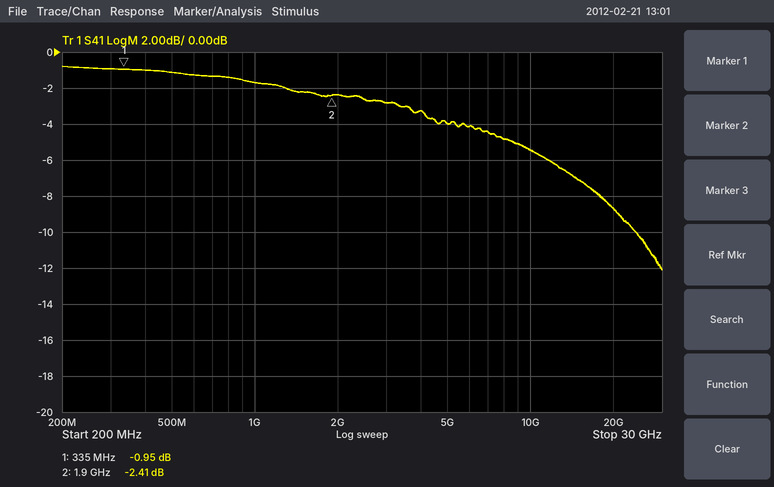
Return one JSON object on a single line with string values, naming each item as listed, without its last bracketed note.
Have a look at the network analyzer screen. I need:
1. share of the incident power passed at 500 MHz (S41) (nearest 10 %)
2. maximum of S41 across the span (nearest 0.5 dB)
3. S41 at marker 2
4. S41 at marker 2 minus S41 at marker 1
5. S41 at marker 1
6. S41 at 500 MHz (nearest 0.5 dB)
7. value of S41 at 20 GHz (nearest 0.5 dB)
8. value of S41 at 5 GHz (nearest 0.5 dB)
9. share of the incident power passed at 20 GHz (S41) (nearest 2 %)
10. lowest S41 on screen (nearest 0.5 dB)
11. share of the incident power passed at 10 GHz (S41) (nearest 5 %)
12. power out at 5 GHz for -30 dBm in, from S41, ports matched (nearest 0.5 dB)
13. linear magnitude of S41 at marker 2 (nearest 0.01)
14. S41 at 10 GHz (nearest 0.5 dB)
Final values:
{"share of the incident power passed at 500 MHz (S41)": "80 %", "maximum of S41 across the span": "-1.0 dB", "S41 at marker 2": "-2.41 dB", "S41 at marker 2 minus S41 at marker 1": "-1.46 dB", "S41 at marker 1": "-0.95 dB", "S41 at 500 MHz": "-1.0 dB", "value of S41 at 20 GHz": "-8.5 dB", "value of S41 at 5 GHz": "-4.0 dB", "share of the incident power passed at 20 GHz (S41)": "14 %", "lowest S41 on screen": "-12.0 dB", "share of the incident power passed at 10 GHz (S41)": "30 %", "power out at 5 GHz for -30 dBm in, from S41, ports matched": "-34.0 dBm", "linear magnitude of S41 at marker 2": "0.76", "S41 at 10 GHz": "-5.5 dB"}
